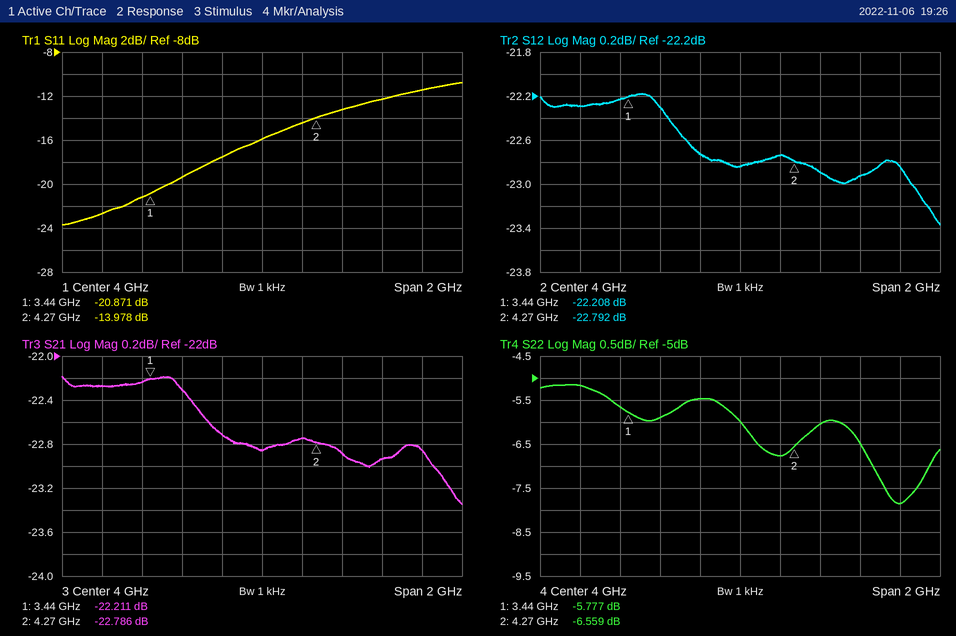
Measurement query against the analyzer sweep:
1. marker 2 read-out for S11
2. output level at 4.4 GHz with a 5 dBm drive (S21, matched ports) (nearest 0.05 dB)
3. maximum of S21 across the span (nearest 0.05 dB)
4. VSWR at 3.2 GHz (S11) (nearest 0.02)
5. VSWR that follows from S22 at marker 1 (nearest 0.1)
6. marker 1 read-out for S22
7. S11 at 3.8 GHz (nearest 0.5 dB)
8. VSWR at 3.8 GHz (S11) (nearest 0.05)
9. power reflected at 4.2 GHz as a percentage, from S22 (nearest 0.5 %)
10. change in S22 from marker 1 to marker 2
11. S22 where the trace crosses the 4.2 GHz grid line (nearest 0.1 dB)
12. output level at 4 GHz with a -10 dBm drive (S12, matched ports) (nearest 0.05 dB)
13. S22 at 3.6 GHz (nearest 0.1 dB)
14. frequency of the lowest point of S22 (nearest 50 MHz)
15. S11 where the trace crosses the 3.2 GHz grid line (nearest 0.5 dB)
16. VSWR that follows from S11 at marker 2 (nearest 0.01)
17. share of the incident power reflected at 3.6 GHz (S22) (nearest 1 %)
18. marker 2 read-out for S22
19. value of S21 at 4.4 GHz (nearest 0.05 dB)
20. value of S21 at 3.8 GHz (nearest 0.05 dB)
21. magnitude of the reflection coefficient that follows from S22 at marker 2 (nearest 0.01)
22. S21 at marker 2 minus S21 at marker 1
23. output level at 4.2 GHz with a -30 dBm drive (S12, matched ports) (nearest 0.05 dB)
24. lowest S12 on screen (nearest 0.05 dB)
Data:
-13.978 dB
-17.90 dBm
-22.20 dB
1.16
3.1
-5.777 dB
-17.5 dB
1.30
21.0 %
-0.782 dB
-6.8 dB
-32.85 dBm
-5.9 dB
4.80 GHz
-22.5 dB
1.50
26 %
-6.559 dB
-22.90 dB
-22.70 dB
0.47
-0.575 dB
-52.75 dBm
-23.35 dB
